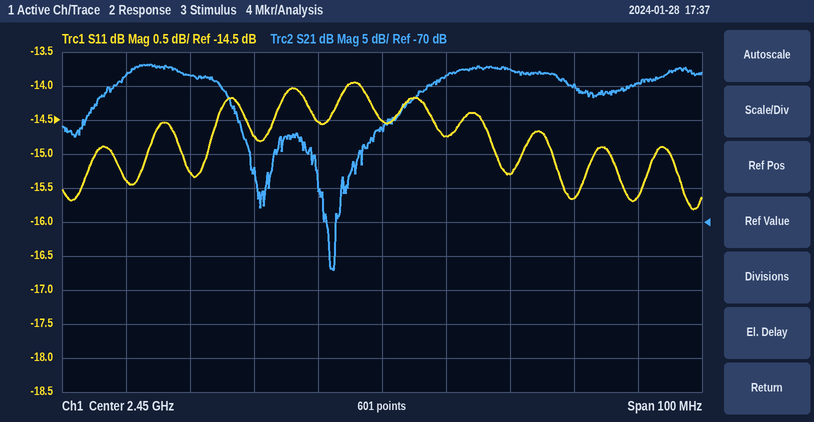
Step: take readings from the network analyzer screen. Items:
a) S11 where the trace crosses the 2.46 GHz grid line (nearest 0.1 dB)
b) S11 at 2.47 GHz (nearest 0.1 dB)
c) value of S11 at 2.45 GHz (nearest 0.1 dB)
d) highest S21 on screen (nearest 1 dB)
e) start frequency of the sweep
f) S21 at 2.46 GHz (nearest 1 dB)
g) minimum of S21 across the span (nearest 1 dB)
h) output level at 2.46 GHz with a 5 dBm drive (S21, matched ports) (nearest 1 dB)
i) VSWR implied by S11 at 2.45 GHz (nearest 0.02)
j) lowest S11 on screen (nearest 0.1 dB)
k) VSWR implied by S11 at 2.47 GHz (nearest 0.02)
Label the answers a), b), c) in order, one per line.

a) -14.7 dB
b) -15.3 dB
c) -14.5 dB
d) -47 dB
e) 2.4 GHz
f) -48 dB
g) -77 dB
h) -43 dBm
i) 1.46
j) -15.8 dB
k) 1.42
